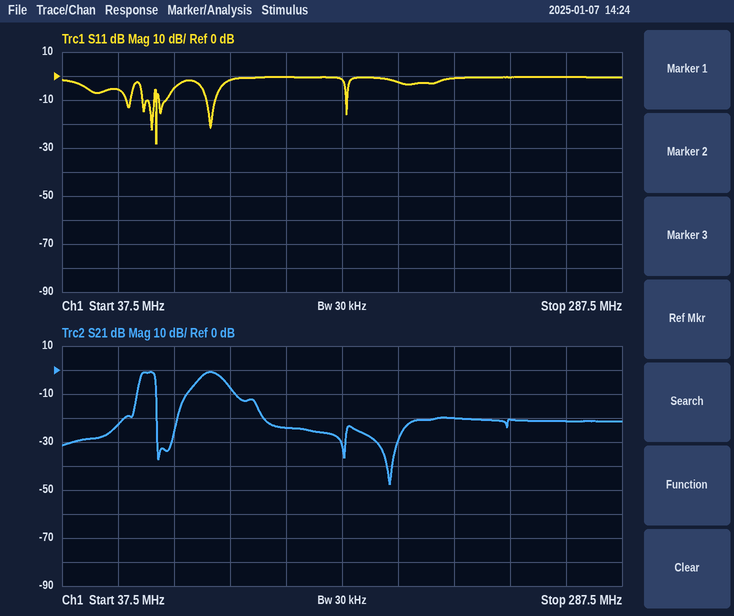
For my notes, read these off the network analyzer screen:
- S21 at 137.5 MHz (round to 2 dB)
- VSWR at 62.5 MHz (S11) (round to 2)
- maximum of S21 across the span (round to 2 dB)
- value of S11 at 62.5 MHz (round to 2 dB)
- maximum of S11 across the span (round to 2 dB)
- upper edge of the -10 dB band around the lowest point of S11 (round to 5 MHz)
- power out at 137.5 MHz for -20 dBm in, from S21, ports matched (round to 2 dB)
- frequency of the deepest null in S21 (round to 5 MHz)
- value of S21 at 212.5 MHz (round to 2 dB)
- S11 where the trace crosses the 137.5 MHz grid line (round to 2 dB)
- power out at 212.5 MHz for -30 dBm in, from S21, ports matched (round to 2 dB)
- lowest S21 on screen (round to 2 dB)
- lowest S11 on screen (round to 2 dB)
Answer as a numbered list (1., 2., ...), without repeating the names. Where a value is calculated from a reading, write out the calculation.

1. -24 dB
2. |Γ| = 10^(-6/20) = 0.5012; VSWR = (1 + 0.5012)/(1 − 0.5012) ≈ 3.01, so 4 to the nearest 2
3. 0 dB
4. -6 dB
5. 0 dB
6. 80 MHz
7. -20 dBm + (-24 dB) = -44 dBm
8. 185 MHz
9. -20 dB
10. 0 dB
11. -30 dBm + (-20 dB) = -50 dBm
12. -48 dB
13. -28 dB
